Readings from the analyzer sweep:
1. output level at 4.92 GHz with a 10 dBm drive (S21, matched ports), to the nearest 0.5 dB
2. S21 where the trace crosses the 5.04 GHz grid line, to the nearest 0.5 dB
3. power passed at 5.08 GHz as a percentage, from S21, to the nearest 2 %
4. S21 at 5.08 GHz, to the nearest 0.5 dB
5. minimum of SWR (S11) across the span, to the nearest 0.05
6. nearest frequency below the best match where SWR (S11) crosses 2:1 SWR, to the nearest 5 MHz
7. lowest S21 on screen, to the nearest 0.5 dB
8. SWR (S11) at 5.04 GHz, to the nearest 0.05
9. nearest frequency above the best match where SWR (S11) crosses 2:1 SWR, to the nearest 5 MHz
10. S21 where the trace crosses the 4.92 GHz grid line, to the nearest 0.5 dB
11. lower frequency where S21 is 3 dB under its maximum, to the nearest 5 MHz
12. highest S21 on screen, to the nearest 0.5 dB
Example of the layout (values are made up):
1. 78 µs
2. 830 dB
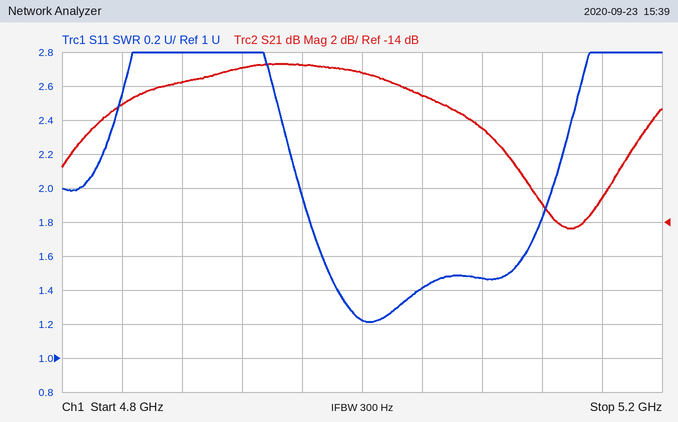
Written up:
1. 5.0 dBm
2. -6.5 dB
3. 14 %
4. -8.5 dB
5. 1.20
6. 4.960 GHz
7. -14.5 dB
8. 1.40
9. 5.125 GHz
10. -5.0 dB
11. 4.830 GHz
12. -4.5 dB
